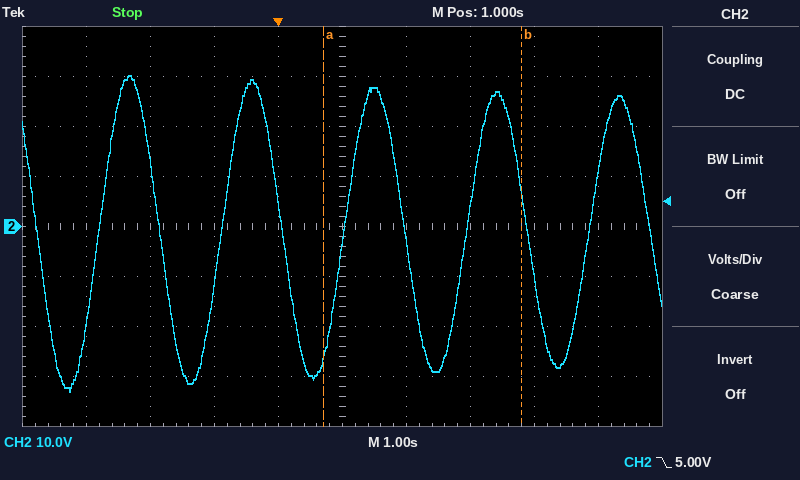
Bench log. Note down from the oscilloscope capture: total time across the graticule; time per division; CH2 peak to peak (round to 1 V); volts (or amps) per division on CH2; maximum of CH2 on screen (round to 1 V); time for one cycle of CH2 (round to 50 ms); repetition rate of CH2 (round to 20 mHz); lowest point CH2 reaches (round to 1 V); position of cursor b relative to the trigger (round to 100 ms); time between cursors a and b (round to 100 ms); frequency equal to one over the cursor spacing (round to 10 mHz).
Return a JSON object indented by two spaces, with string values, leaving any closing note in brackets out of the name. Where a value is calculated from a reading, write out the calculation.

{
  "total time across the graticule": "10 s",
  "time per division": "1 s",
  "CH2 peak to peak": "30 V − (-33 V) = 63 V",
  "volts (or amps) per division on CH2": "10 V",
  "maximum of CH2 on screen": "30 V",
  "time for one cycle of CH2": "1.90 s",
  "repetition rate of CH2": "1 / 1.90 s ≈ 526 mHz, so 520 mHz to the nearest 20 mHz",
  "lowest point CH2 reaches": "-33 V",
  "position of cursor b relative to the trigger": "+3.8 s",
  "time between cursors a and b": "3.1 s",
  "frequency equal to one over the cursor spacing": "1 / 3.1 s ≈ 320 mHz"
}
